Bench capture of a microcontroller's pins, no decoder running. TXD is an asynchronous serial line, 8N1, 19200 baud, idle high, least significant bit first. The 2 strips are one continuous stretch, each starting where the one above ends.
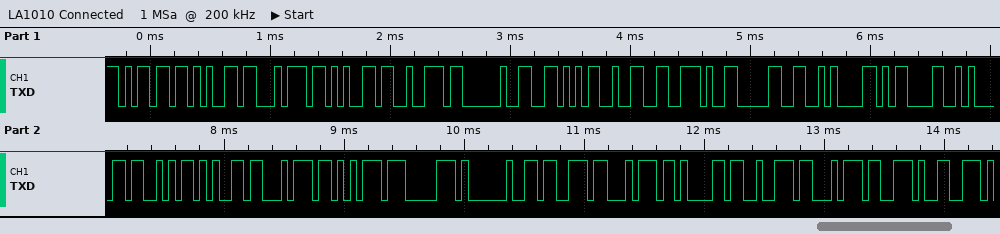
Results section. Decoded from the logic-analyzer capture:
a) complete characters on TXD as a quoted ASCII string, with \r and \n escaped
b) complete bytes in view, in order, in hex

"meter V2.0\n\r\nSetup start."
6D 65 74 65 72 20 56 32 2E 30 0A 0D 0A 53 65 74 75 70 20 73 74 61 72 74 2E
